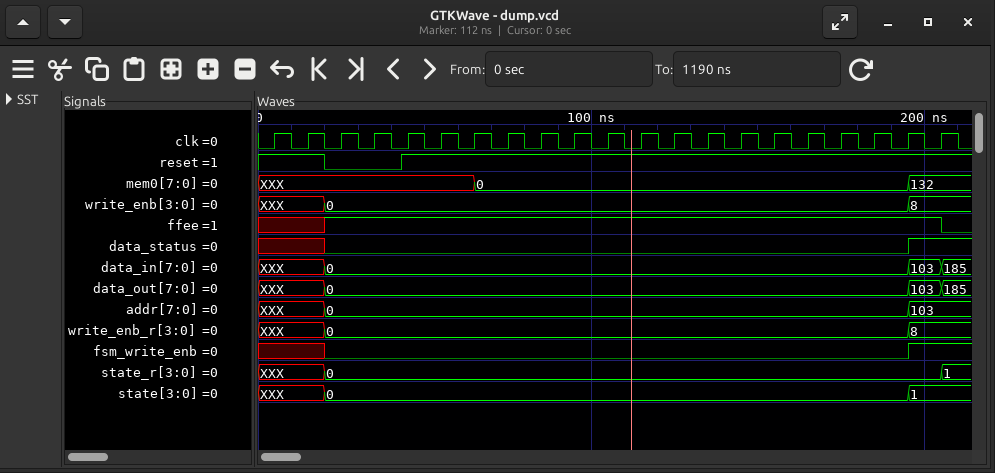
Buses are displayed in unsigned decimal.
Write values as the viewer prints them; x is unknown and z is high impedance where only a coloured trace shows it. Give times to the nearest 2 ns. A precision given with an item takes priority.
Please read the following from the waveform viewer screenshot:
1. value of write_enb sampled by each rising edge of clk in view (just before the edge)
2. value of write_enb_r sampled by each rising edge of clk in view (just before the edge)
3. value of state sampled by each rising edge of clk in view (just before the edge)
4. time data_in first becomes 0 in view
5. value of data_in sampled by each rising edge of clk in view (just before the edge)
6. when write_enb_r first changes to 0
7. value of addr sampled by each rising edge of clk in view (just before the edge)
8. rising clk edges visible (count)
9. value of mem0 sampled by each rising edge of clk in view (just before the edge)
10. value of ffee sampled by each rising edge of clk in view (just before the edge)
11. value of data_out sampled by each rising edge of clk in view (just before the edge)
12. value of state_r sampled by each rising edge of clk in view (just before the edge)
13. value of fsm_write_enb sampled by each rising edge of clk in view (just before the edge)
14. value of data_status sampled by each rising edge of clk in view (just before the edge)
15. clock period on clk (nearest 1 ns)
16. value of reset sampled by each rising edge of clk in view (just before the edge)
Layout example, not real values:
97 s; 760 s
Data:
XXX, XXX, 0, 0, 0, 0, 0, 0, 0, 0, 0, 0, 0, 0, 0, 0, 0, 0, 0, 0, 8; XXX, XXX, 0, 0, 0, 0, 0, 0, 0, 0, 0, 0, 0, 0, 0, 0, 0, 0, 0, 0, 8; XXX, XXX, 0, 0, 0, 0, 0, 0, 0, 0, 0, 0, 0, 0, 0, 0, 0, 0, 0, 0, 1; 20 ns; XXX, XXX, 0, 0, 0, 0, 0, 0, 0, 0, 0, 0, 0, 0, 0, 0, 0, 0, 0, 0, 103; 20 ns; XXX, XXX, 0, 0, 0, 0, 0, 0, 0, 0, 0, 0, 0, 0, 0, 0, 0, 0, 0, 0, 103; 21; XXX, XXX, XXX, XXX, XXX, XXX, XXX, 0, 0, 0, 0, 0, 0, 0, 0, 0, 0, 0, 0, 0, 132; x x 1 1 1 1 1 1 1 1 1 1 1 1 1 1 1 1 1 1 1; XXX, XXX, 0, 0, 0, 0, 0, 0, 0, 0, 0, 0, 0, 0, 0, 0, 0, 0, 0, 0, 103; XXX, XXX, 0, 0, 0, 0, 0, 0, 0, 0, 0, 0, 0, 0, 0, 0, 0, 0, 0, 0, 0; x x 0 0 0 0 0 0 0 0 0 0 0 0 0 0 0 0 0 0 1; x x 0 0 0 0 0 0 0 0 0 0 0 0 0 0 0 0 0 0 1; 10 ns; 1 1 0 0 1 1 1 1 1 1 1 1 1 1 1 1 1 1 1 1 1
